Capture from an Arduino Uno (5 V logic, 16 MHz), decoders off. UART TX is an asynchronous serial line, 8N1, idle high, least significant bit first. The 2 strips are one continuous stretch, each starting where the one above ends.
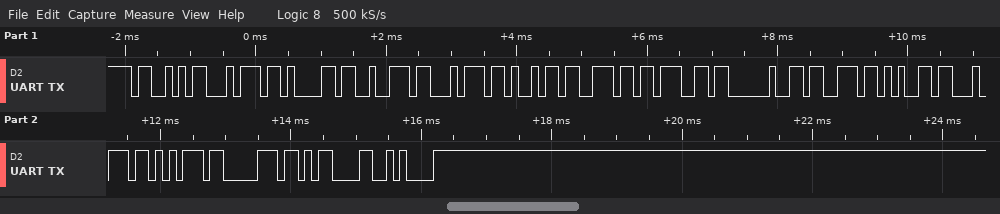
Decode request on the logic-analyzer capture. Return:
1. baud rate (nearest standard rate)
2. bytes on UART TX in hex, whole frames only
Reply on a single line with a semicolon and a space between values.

9600 baud; 0x53 0x74 0x61 0x72 0x74 0x69 0x6E 0x67 0x20 0x73 0x65 0x74 0x75 0x70 0x0D 0x0A
